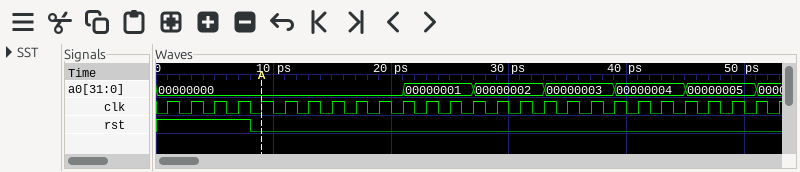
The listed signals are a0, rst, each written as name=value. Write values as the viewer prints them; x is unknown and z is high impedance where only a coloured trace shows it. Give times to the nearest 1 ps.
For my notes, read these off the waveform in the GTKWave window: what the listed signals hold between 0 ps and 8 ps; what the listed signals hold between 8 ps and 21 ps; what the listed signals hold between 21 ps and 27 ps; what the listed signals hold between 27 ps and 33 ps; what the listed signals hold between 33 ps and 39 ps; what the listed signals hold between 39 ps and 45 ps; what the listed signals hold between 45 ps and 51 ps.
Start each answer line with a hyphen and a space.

- a0=00000000, rst=1
- a0=00000000, rst=0
- a0=00000001, rst=0
- a0=00000002, rst=0
- a0=00000003, rst=0
- a0=00000004, rst=0
- a0=00000005, rst=0
